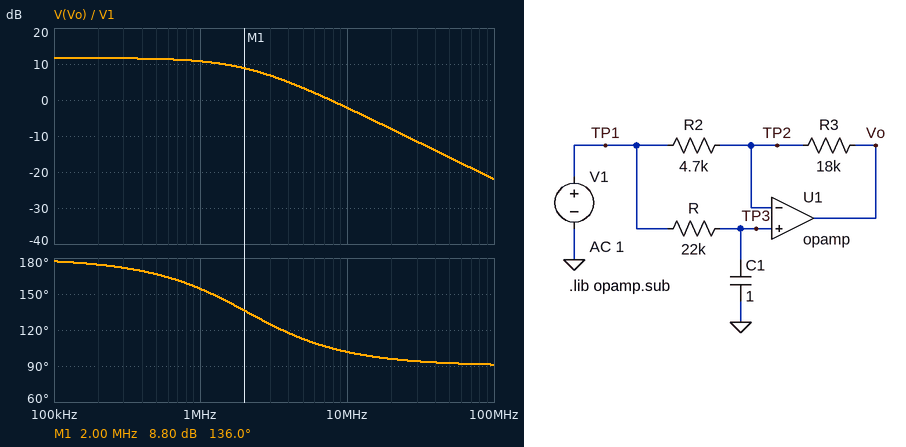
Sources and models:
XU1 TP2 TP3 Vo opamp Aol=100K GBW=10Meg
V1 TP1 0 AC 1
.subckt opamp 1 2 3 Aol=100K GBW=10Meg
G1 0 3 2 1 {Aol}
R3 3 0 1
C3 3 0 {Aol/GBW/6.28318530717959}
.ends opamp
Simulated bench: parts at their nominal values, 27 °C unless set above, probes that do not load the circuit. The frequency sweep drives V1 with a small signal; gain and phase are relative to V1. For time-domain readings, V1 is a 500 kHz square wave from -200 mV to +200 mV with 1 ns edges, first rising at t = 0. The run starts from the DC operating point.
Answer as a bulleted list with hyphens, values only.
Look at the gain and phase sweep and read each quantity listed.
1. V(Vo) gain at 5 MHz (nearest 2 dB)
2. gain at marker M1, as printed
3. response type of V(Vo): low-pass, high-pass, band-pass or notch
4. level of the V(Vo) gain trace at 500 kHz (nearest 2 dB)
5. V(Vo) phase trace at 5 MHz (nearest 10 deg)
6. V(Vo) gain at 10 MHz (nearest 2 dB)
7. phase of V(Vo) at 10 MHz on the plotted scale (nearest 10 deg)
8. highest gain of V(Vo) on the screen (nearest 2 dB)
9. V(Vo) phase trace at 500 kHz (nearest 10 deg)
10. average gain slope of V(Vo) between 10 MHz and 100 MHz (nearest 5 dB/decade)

- 4 dB
- 8.80 dB
- low-pass
- 12 dB
- 110 deg
- -2 dB
- 100 deg
- 12 dB
- 170 deg
- -20 dB/decade
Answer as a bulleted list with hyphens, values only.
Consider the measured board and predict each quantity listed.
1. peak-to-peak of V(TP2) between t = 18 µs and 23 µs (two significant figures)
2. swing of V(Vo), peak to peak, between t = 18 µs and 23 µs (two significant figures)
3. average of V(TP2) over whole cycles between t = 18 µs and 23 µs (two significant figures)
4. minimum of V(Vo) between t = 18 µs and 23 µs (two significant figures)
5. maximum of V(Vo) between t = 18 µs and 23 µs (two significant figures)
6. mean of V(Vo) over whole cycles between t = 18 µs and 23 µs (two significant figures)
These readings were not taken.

- 630 mV
- 1.5 V
- -200 mV
- -1.7 V
- -200 mV
- -970 mV
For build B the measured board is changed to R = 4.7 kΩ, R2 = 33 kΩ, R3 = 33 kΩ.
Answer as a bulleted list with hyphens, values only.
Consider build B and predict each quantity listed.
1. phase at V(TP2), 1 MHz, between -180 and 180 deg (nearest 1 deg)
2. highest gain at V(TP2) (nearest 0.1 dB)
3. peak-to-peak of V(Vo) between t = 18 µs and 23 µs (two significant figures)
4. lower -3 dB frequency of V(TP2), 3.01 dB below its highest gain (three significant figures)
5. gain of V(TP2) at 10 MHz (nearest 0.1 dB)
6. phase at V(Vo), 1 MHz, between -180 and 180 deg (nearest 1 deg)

- 79 deg
- -6.0 dB
- 400 mV
- 5.00 MHz
- -7.0 dB
- 169 deg
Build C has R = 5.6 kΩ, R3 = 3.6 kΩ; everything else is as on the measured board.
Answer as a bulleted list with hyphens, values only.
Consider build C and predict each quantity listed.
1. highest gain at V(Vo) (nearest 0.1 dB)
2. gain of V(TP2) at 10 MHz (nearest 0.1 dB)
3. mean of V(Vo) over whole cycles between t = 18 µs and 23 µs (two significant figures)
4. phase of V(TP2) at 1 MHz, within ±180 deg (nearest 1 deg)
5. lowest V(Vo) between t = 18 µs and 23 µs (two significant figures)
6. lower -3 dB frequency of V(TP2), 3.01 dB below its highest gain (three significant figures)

- -2.3 dB
- -8.5 dB
- -350 mV
- 80 deg
- -510 mV
- 5.66 MHz
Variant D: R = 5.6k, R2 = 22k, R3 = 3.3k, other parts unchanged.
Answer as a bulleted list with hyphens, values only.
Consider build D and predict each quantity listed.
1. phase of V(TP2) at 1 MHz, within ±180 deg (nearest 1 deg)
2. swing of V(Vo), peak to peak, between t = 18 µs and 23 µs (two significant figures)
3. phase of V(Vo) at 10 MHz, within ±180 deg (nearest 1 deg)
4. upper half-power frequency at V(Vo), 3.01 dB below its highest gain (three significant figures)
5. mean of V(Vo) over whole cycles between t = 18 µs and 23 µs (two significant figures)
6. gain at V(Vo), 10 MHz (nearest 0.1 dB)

- 83 deg
- 60 mV
- 131 deg
- 8.70 MHz
- -230 mV
- -20.1 dB
